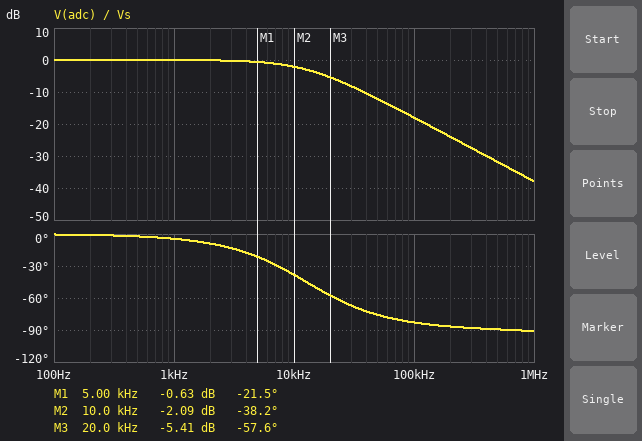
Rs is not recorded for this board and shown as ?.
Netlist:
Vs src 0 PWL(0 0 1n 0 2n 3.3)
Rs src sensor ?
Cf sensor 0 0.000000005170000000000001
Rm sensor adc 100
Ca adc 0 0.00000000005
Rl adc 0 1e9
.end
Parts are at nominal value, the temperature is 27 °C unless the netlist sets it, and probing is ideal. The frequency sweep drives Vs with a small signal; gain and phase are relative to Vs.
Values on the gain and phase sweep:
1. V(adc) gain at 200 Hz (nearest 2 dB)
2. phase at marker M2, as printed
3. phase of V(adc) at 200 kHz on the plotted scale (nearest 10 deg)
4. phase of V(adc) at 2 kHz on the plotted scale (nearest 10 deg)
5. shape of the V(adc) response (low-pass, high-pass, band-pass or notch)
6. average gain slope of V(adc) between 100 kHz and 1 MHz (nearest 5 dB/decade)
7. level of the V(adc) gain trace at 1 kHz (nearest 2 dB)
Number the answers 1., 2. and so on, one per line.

1. 0 dB
2. -38.2 deg
3. -90 deg
4. -10 deg
5. low-pass
6. -20 dB/decade
7. 0 dB
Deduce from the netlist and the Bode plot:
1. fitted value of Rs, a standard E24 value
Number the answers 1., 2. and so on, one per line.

1. 2.4 kΩ
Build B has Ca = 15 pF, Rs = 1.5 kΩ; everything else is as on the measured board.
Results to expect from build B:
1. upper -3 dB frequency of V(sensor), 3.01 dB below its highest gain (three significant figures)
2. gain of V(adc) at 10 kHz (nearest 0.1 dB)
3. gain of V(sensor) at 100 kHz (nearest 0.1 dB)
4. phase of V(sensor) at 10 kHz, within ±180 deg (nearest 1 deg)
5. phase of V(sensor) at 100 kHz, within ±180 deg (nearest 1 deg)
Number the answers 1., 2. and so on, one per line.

1. 20.5 kHz
2. -0.9 dB
3. -14.0 dB
4. -26 deg
5. -78 deg
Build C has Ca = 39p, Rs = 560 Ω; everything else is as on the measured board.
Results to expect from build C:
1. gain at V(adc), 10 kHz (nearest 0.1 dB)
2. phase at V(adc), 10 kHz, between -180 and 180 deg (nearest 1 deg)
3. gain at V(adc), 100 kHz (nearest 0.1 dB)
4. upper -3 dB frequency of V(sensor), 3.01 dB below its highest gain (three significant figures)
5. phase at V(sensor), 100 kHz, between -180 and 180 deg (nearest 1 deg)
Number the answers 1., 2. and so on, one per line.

1. -0.1 dB
2. -10 deg
3. -6.4 dB
4. 54.6 kHz
5. -61 deg
